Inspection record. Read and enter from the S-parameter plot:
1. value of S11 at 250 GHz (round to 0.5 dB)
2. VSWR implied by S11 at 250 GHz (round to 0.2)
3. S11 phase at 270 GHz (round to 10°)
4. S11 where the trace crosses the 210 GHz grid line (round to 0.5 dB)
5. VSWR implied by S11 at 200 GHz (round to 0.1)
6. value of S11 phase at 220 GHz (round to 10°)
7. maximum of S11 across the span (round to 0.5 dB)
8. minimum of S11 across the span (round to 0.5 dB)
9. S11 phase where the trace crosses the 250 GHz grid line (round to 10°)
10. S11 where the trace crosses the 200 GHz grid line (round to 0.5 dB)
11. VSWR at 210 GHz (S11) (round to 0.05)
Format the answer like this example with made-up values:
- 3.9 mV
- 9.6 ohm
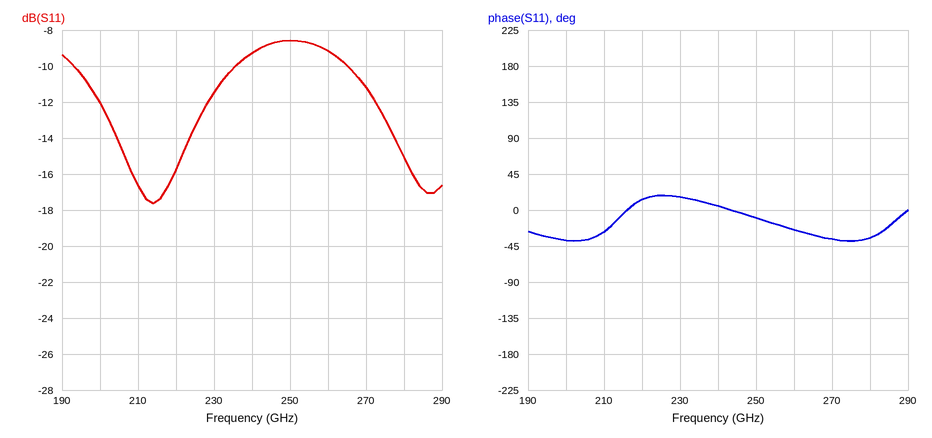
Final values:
- -8.5 dB
- 2.2
- -40°
- -16.5 dB
- 1.7
- 10°
- -8.5 dB
- -17.5 dB
- -10°
- -12.0 dB
- 1.35
